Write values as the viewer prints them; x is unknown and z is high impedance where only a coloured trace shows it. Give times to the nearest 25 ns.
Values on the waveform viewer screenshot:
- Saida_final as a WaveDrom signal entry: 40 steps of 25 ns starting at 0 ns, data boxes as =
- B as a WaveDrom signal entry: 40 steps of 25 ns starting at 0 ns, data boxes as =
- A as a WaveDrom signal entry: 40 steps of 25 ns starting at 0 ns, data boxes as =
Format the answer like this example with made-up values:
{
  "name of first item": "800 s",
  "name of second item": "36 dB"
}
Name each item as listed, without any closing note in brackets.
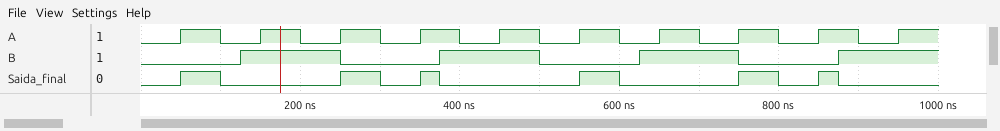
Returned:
{
  "Saida_final as a WaveDrom signal entry: 40 steps of 25 ns starting at 0 ns, data boxes as =": "{name: 'Saida_final', wave: '0.1.0.....1.0.10......1.0.....1.0.10....'}",
  "B as a WaveDrom signal entry: 40 steps of 25 ns starting at 0 ns, data boxes as =": "{name: 'B', wave: '0....1....0....1....0....1....0....1....'}",
  "A as a WaveDrom signal entry: 40 steps of 25 ns starting at 0 ns, data boxes as =": "{name: 'A', wave: '0.1.0.1.0.1.0.1.0.1.0.1.0.1.0.1.0.1.0.1.'}"
}
